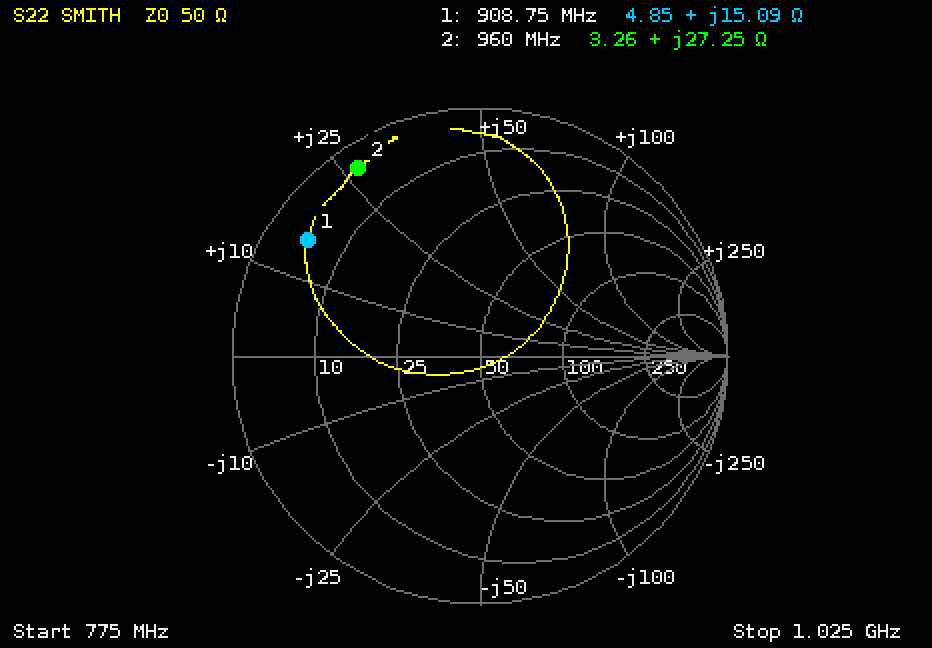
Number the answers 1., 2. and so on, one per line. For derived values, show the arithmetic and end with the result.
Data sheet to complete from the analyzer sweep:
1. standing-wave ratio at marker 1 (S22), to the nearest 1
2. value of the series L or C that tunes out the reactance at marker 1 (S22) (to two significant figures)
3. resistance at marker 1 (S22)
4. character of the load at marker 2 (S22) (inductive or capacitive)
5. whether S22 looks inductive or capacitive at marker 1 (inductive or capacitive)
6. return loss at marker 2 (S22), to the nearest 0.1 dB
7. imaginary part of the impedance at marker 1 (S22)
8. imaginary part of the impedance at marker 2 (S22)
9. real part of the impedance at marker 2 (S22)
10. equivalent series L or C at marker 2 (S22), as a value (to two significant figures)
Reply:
1. 11
2. C = 1/(2π × 908.75 MHz × 15.09 Ω) ≈ 12 pF
3. 4.85 Ω
4. inductive
5. inductive
6. 0.9 dB
7. +15.09 Ω
8. +27.25 Ω
9. 3.26 Ω
10. L = 27.25 Ω/(2π × 960 MHz) ≈ 4.5 nH
